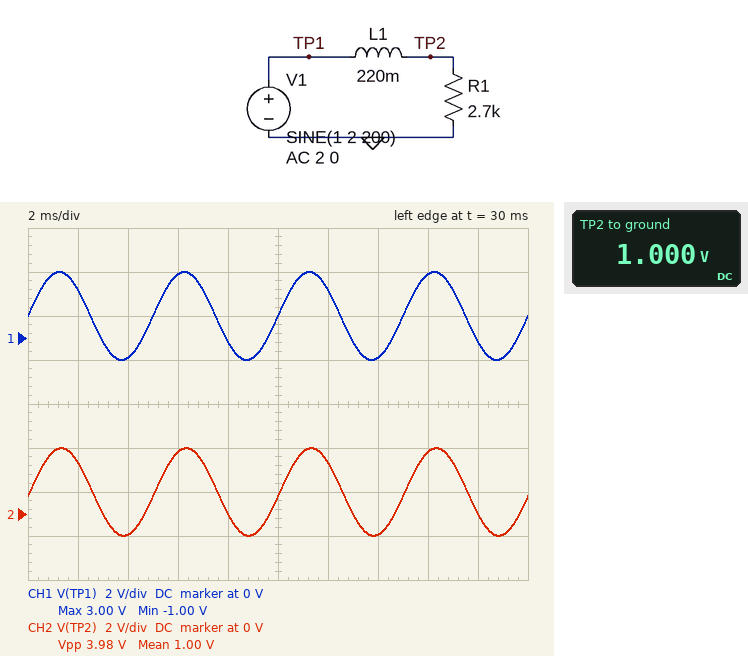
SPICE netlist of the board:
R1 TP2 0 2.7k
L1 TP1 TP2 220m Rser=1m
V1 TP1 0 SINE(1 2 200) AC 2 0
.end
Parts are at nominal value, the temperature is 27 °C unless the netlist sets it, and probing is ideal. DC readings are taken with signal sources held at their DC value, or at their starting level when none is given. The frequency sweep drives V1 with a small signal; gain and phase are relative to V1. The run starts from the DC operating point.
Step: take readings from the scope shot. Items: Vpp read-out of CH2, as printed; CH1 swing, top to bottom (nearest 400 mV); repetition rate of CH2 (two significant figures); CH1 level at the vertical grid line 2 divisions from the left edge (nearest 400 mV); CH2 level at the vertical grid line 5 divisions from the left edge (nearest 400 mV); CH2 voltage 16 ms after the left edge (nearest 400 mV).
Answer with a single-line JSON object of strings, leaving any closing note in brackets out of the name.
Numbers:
{"Vpp read-out of CH2, as printed": "3.98 V", "CH1 swing, top to bottom": "4.0 V", "repetition rate of CH2": "200 Hz", "CH1 level at the vertical grid line 2 divisions from the left edge": "-800 mV", "CH2 level at the vertical grid line 5 divisions from the left edge": "800 mV", "CH2 voltage 16 ms after the left edge": "2.8 V"}
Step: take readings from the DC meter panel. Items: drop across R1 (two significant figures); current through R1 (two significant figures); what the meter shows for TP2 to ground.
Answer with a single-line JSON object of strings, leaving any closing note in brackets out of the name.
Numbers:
{"drop across R1": "1.0 V", "current through R1": "370 µA", "what the meter shows for TP2 to ground": "1.000 V"}
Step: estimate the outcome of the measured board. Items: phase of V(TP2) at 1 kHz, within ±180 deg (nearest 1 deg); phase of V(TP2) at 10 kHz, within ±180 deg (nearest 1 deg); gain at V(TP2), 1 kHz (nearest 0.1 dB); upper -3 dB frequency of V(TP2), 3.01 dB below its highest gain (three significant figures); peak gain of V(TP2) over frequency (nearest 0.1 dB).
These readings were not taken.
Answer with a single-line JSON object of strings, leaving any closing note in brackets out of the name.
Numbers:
{"phase of V(TP2) at 1 kHz, within ±180 deg": "-27 deg", "phase of V(TP2) at 10 kHz, within ±180 deg": "-79 deg", "gain at V(TP2), 1 kHz": "-1.0 dB", "upper -3 dB frequency of V(TP2), 3.01 dB below its highest gain": "1.95 kHz", "peak gain of V(TP2) over frequency": "0 dB"}
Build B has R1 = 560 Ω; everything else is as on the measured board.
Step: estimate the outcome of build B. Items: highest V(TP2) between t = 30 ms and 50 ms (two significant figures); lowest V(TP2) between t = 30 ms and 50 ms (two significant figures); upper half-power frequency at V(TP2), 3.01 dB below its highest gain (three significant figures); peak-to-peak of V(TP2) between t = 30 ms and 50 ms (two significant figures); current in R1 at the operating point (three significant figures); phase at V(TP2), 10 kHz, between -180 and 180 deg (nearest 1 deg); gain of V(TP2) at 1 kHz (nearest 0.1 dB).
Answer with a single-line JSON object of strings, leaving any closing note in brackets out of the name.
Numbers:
{"highest V(TP2) between t = 30 ms and 50 ms": "2.8 V", "lowest V(TP2) between t = 30 ms and 50 ms": "-790 mV", "upper half-power frequency at V(TP2), 3.01 dB below its highest gain": "405 Hz", "peak-to-peak of V(TP2) between t = 30 ms and 50 ms": "3.6 V", "current in R1 at the operating point": "1.79 mA", "phase at V(TP2), 10 kHz, between -180 and 180 deg": "-88 deg", "gain of V(TP2) at 1 kHz": "-8.5 dB"}
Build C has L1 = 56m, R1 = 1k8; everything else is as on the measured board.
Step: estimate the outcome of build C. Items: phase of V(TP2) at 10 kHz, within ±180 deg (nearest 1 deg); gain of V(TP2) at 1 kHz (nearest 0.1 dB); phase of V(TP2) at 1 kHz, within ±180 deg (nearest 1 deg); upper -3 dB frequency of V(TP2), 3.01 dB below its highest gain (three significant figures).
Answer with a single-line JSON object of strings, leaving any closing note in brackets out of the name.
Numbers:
{"phase of V(TP2) at 10 kHz, within ±180 deg": "-63 deg", "gain of V(TP2) at 1 kHz": "-0.2 dB", "phase of V(TP2) at 1 kHz, within ±180 deg": "-11 deg", "upper -3 dB frequency of V(TP2), 3.01 dB below its highest gain": "5.12 kHz"}
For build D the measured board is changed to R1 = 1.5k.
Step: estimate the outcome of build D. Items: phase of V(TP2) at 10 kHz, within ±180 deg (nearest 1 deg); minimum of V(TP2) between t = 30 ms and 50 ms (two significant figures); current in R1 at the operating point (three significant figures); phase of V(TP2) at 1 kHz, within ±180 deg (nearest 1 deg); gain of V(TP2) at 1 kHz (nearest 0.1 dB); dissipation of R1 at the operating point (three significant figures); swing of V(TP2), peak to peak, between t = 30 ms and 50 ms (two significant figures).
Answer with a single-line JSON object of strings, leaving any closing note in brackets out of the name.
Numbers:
{"phase of V(TP2) at 10 kHz, within ±180 deg": "-84 deg", "minimum of V(TP2) between t = 30 ms and 50 ms": "-970 mV", "current in R1 at the operating point": "667 µA", "phase of V(TP2) at 1 kHz, within ±180 deg": "-43 deg", "gain of V(TP2) at 1 kHz": "-2.7 dB", "dissipation of R1 at the operating point": "667 µW", "swing of V(TP2), peak to peak, between t = 30 ms and 50 ms": "3.9 V"}
